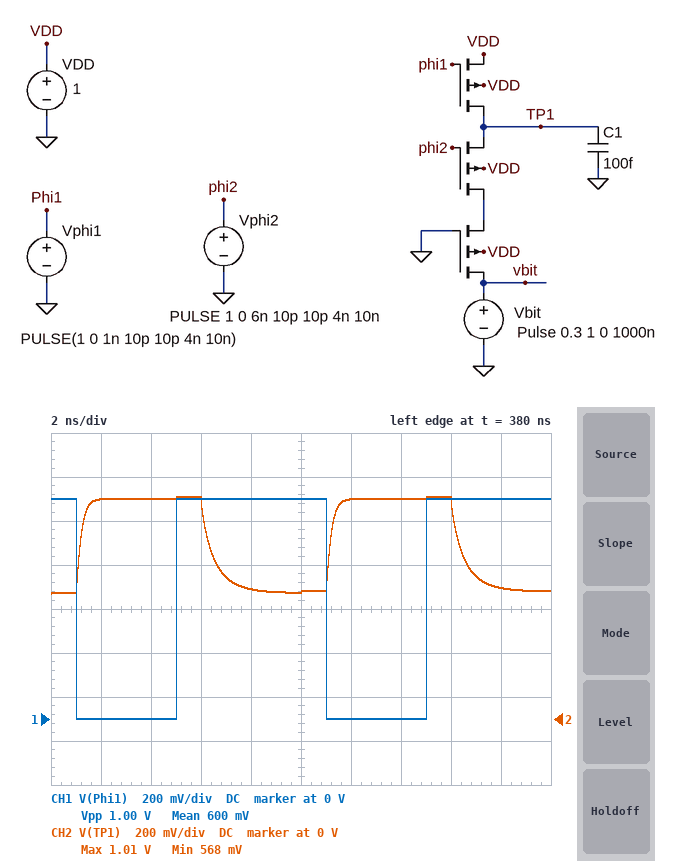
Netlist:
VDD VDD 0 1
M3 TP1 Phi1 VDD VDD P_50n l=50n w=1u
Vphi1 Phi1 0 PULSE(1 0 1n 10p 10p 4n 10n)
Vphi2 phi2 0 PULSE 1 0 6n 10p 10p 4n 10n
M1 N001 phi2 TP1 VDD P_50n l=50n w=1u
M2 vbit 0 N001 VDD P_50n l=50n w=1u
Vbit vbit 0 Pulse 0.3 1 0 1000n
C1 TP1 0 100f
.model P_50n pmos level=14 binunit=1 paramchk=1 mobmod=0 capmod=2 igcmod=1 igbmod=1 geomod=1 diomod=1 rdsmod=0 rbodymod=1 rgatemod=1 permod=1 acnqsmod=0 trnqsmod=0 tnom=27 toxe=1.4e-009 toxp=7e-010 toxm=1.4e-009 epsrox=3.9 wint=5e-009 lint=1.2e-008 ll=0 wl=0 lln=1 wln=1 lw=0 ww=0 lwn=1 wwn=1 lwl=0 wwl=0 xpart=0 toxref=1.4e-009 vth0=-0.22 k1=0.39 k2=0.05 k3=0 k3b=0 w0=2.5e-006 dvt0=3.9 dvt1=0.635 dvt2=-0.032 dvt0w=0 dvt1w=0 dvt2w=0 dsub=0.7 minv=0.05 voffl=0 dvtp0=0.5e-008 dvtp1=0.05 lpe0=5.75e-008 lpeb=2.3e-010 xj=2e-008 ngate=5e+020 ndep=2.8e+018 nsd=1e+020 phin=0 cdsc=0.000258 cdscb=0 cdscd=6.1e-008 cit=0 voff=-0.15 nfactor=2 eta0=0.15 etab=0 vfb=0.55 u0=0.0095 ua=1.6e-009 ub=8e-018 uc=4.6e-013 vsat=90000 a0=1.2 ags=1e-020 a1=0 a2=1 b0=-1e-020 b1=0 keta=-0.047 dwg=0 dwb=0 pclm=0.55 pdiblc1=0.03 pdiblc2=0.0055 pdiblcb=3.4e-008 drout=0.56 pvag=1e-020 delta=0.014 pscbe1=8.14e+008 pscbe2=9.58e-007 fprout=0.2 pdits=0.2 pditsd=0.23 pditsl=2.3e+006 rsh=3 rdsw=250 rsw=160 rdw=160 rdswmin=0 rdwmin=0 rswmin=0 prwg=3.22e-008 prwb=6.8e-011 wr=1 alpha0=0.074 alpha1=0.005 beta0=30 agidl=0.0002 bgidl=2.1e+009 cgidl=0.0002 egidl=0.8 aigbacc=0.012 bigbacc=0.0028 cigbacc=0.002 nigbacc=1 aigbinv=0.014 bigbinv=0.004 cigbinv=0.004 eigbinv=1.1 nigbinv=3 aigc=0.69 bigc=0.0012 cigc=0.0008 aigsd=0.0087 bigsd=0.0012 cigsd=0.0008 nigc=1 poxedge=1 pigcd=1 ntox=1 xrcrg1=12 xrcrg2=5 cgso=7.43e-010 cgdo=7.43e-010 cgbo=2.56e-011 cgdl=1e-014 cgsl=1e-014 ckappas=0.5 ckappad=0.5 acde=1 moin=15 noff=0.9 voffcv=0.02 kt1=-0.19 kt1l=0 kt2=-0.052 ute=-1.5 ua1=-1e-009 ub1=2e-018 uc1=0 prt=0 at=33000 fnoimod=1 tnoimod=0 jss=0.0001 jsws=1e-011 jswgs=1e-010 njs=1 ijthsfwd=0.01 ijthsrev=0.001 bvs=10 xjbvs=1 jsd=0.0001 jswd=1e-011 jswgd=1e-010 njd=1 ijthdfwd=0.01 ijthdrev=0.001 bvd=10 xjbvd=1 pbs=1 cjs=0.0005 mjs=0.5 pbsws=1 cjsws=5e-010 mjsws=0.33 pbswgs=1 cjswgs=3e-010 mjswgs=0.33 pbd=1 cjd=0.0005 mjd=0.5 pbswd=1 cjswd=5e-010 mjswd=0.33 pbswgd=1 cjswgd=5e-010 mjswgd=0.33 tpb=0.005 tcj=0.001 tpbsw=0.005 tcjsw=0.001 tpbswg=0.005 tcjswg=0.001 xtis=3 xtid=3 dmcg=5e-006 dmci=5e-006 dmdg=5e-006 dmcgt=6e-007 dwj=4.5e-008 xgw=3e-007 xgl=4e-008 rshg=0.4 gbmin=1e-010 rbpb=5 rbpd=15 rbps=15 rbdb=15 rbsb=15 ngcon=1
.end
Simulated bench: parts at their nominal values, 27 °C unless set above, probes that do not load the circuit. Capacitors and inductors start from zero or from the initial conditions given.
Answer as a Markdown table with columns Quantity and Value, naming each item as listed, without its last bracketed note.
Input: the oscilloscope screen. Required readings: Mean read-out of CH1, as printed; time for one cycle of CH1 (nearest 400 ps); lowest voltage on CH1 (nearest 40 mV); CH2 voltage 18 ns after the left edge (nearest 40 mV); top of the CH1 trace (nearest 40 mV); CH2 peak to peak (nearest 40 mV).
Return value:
| Quantity | Value |
|---|---|
| Mean read-out of CH1, as printed | 600 mV |
| time for one cycle of CH1 | 10.0 ns |
| lowest voltage on CH1 | 0 V |
| CH2 voltage 18 ns after the left edge | 600 mV |
| top of the CH1 trace | 1.00 V |
| CH2 peak to peak | 440 mV |
